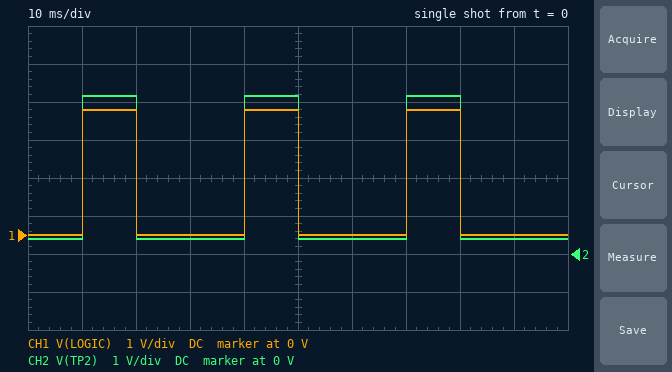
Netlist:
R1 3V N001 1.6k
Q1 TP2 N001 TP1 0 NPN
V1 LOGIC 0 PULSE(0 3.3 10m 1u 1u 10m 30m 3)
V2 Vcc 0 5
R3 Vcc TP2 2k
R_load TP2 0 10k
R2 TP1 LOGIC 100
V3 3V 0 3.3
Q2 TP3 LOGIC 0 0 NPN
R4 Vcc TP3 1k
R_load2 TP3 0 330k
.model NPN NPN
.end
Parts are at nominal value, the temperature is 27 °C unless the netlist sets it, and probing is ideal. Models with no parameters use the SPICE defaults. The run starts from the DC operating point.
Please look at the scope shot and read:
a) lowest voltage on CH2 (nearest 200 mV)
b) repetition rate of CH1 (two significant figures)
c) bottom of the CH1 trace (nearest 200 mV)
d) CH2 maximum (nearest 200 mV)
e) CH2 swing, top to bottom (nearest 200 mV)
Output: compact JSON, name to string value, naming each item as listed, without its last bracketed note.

{"lowest voltage on CH2": "400 mV", "repetition rate of CH1": "33 Hz", "bottom of the CH1 trace": "0 V", "CH2 maximum": "4.2 V", "CH2 swing, top to bottom": "3.8 V"}
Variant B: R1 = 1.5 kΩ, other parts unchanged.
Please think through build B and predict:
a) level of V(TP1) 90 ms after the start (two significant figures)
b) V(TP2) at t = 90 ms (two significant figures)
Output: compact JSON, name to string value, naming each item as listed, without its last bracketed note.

{"level of V(TP1) 90 ms after the start": "370 mV", "V(TP2) at t = 90 ms": "400 mV"}
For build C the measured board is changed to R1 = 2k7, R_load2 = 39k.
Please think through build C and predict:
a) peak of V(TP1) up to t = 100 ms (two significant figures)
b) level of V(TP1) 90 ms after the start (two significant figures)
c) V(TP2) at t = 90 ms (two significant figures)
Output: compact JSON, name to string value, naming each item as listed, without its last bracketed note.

{"peak of V(TP1) up to t = 100 ms": "3.3 V", "level of V(TP1) 90 ms after the start": "310 mV", "V(TP2) at t = 90 ms": "350 mV"}
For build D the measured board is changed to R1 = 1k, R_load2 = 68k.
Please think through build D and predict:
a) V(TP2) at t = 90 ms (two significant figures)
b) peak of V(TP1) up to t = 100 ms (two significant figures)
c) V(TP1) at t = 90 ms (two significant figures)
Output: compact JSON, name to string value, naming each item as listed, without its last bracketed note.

{"V(TP2) at t = 90 ms": "460 mV", "peak of V(TP1) up to t = 100 ms": "3.3 V", "V(TP1) at t = 90 ms": "430 mV"}
